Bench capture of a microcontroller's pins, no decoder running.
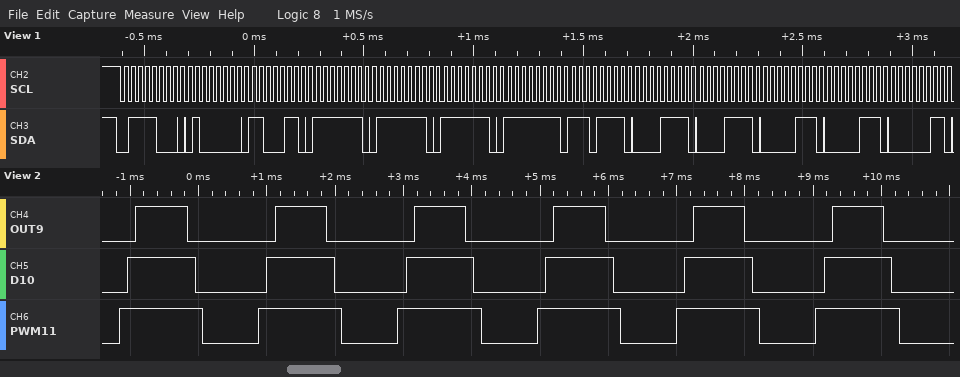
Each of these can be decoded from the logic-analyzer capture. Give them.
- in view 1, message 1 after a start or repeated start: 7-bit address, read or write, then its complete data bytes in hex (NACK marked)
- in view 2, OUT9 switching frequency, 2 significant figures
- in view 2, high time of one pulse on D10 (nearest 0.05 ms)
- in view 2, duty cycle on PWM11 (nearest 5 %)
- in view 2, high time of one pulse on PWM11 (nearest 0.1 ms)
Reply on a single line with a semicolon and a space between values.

0x3C write: 40 C6 FE FE FE FF EF 0F 0F 07 07 03; 490 Hz; 1.00 ms; 60 %; 1.2 ms
